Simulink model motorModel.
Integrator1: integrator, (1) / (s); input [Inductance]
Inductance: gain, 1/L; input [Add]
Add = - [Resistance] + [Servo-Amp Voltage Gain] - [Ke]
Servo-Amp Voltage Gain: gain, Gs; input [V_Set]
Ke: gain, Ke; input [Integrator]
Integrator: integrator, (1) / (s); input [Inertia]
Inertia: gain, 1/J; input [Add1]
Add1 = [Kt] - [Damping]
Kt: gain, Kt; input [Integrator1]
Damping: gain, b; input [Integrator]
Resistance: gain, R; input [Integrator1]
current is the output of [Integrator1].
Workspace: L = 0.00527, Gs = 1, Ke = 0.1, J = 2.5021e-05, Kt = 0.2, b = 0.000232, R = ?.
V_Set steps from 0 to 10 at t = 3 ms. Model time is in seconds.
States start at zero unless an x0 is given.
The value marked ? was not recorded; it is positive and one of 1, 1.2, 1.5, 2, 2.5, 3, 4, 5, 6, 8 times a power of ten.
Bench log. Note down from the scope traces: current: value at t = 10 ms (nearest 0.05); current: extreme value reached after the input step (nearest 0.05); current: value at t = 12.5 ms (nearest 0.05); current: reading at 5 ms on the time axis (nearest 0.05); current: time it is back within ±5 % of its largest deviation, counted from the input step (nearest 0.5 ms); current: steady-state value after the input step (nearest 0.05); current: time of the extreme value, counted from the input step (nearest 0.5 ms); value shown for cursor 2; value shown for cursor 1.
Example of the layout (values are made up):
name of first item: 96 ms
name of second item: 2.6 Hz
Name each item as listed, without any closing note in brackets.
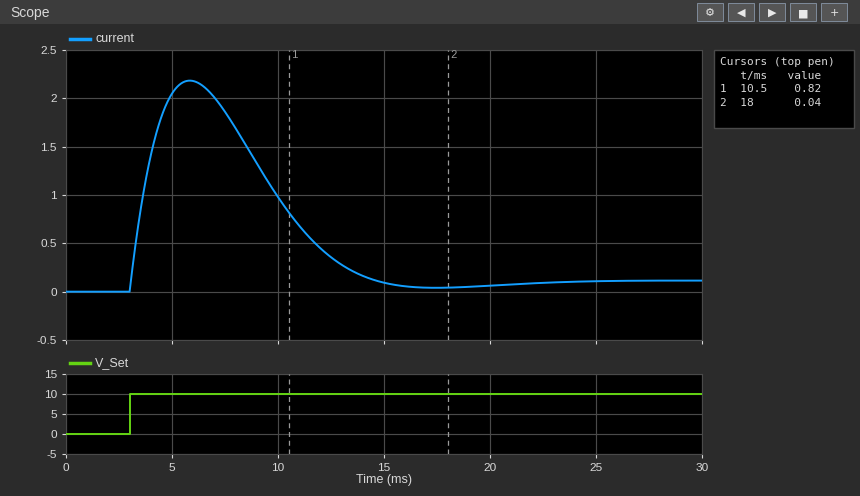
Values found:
current: value at t = 10 ms: 1.00
current: extreme value reached after the input step: 2.20
current: value at t = 12.5 ms: 0.35
current: reading at 5 ms on the time axis: 2.05
current: time it is back within ±5 % of its largest deviation, counted from the input step: 10.5 ms
current: steady-state value after the input step: 0.10
current: time of the extreme value, counted from the input step: 3.0 ms
value shown for cursor 2: 0.04
value shown for cursor 1: 0.82
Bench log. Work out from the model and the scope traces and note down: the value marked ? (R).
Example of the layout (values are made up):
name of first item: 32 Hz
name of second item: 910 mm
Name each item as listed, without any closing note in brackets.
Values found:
the value marked ?: 3
